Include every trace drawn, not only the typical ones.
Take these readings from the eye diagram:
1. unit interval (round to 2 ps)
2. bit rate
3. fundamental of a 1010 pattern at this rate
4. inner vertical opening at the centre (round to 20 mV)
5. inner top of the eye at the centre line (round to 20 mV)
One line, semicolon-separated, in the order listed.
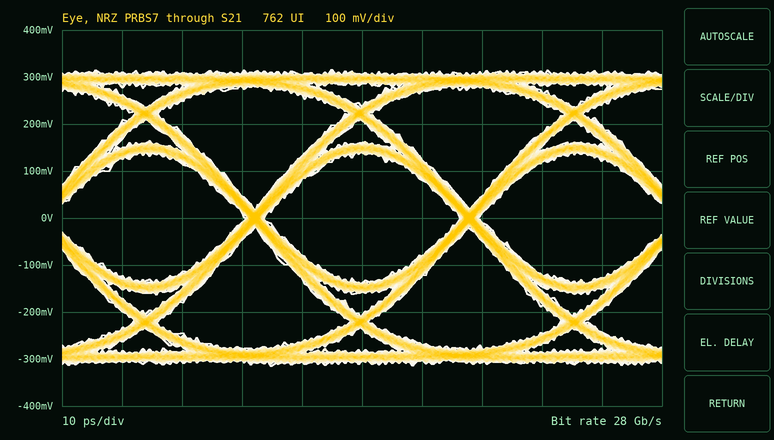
36 ps; 28 Gb/s; 14 GHz; 280 mV; 140 mV
